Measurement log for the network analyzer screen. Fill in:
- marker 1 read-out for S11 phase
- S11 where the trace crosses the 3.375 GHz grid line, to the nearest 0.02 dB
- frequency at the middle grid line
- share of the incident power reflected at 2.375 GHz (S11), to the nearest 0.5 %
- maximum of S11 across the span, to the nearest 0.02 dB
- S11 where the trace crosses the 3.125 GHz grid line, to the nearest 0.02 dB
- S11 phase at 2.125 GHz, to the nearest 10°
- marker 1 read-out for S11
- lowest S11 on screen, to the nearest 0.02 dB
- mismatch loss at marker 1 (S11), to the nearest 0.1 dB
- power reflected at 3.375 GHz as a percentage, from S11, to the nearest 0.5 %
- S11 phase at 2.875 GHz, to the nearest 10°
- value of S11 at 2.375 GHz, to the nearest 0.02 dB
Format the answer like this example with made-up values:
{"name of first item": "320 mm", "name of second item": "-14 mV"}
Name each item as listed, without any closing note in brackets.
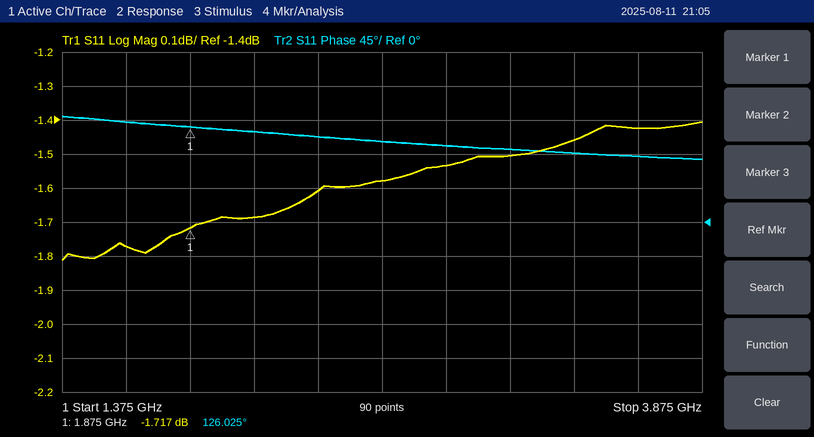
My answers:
{"marker 1 read-out for S11 phase": "126.025°", "S11 where the trace crosses the 3.375 GHz grid line, to the nearest 0.02 dB": "-1.46 dB", "frequency at the middle grid line": "2.625 GHz", "share of the incident power reflected at 2.375 GHz (S11), to the nearest 0.5 %": "69.0 %", "maximum of S11 across the span, to the nearest 0.02 dB": "-1.40 dB", "S11 where the trace crosses the 3.125 GHz grid line, to the nearest 0.02 dB": "-1.50 dB", "S11 phase at 2.125 GHz, to the nearest 10°": "120°", "marker 1 read-out for S11": "-1.717 dB", "lowest S11 on screen, to the nearest 0.02 dB": "-1.82 dB", "mismatch loss at marker 1 (S11), to the nearest 0.1 dB": "4.9 dB", "power reflected at 3.375 GHz as a percentage, from S11, to the nearest 0.5 %": "71.5 %", "S11 phase at 2.875 GHz, to the nearest 10°": "100°", "value of S11 at 2.375 GHz, to the nearest 0.02 dB": "-1.60 dB"}
